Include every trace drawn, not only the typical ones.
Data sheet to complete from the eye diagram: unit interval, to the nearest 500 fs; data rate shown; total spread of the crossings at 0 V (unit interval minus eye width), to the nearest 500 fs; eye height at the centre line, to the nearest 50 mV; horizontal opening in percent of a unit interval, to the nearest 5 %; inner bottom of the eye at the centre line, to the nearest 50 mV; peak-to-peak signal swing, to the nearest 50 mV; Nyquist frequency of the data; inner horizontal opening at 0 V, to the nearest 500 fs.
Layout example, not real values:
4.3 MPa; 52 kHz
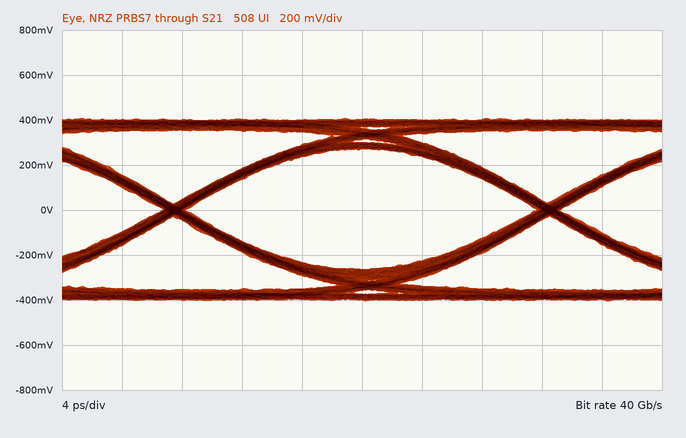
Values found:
25.0 ps; 40 Gb/s; 1.5 ps; 550 mV; 95 %; -250 mV; 800 mV; 20 GHz; 23.5 ps
